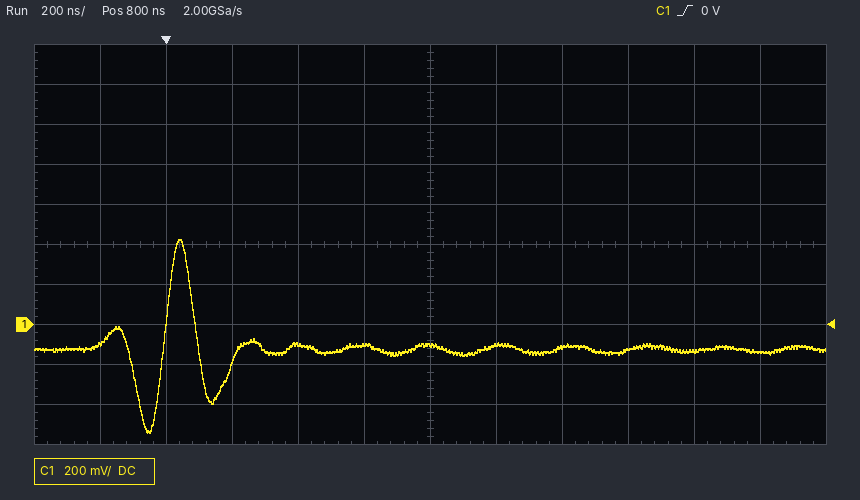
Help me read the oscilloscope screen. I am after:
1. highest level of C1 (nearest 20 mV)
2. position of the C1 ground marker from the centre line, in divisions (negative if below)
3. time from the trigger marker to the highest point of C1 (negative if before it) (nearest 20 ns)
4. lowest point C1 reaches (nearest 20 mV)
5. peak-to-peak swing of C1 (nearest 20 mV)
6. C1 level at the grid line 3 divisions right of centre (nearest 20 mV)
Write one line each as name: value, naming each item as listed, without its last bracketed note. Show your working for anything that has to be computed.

highest level of C1: 420 mV
position of the C1 ground marker from the centre line, in divisions: -2.0 div
time from the trigger marker to the highest point of C1 (negative if before it): +40 ns
lowest point C1 reaches: -540 mV
peak-to-peak swing of C1: 420 mV − (-540 mV) = 960 mV
C1 level at the grid line 3 divisions right of centre: -120 mV
